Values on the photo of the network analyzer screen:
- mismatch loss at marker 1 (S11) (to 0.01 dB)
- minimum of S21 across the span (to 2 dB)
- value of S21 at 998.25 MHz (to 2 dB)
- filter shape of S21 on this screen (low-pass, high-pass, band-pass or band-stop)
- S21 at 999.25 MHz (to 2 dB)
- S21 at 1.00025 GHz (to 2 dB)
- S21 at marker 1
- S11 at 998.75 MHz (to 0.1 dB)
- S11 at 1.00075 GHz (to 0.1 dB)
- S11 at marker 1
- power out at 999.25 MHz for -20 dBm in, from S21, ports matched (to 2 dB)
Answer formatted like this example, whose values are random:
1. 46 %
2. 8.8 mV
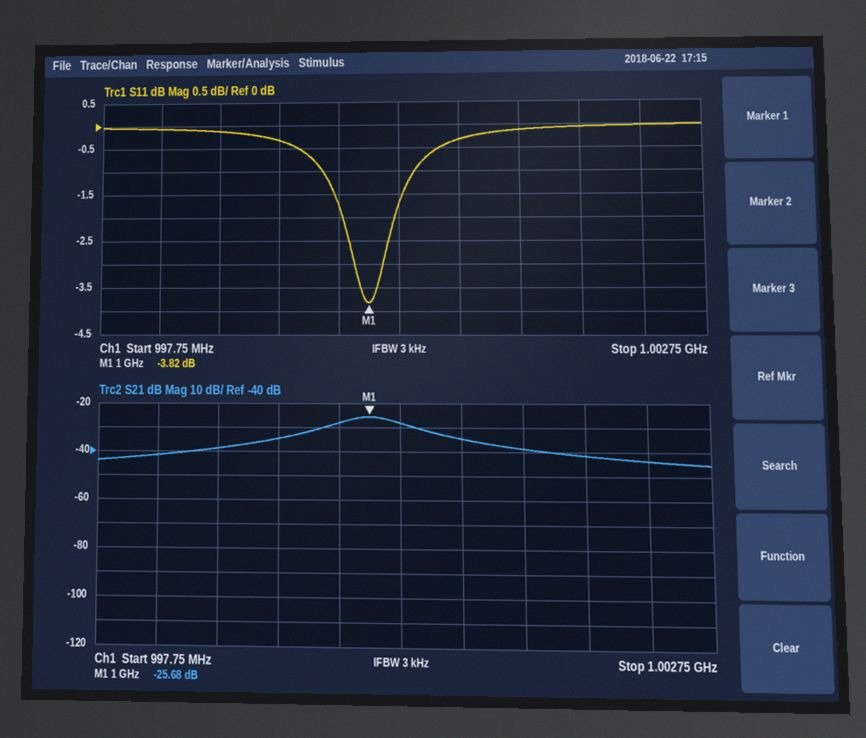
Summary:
1. 2.33 dB
2. -46 dB
3. -42 dB
4. band-pass
5. -34 dB
6. -28 dB
7. -25.68 dB
8. -0.1 dB
9. -0.3 dB
10. -3.82 dB
11. -54 dBm
